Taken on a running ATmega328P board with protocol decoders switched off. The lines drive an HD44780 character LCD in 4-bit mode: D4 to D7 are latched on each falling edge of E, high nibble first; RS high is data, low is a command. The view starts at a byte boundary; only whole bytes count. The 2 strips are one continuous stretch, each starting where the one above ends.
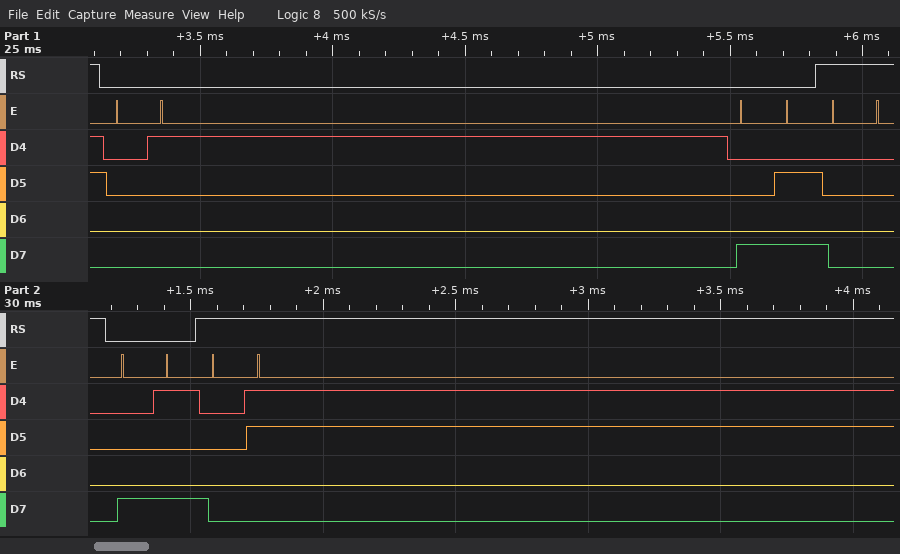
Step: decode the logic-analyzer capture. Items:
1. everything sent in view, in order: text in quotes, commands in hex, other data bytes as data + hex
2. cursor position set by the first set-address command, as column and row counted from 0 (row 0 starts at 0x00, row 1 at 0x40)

0x01 0x8A data 00 0x89 data 03
column 10, row 0
